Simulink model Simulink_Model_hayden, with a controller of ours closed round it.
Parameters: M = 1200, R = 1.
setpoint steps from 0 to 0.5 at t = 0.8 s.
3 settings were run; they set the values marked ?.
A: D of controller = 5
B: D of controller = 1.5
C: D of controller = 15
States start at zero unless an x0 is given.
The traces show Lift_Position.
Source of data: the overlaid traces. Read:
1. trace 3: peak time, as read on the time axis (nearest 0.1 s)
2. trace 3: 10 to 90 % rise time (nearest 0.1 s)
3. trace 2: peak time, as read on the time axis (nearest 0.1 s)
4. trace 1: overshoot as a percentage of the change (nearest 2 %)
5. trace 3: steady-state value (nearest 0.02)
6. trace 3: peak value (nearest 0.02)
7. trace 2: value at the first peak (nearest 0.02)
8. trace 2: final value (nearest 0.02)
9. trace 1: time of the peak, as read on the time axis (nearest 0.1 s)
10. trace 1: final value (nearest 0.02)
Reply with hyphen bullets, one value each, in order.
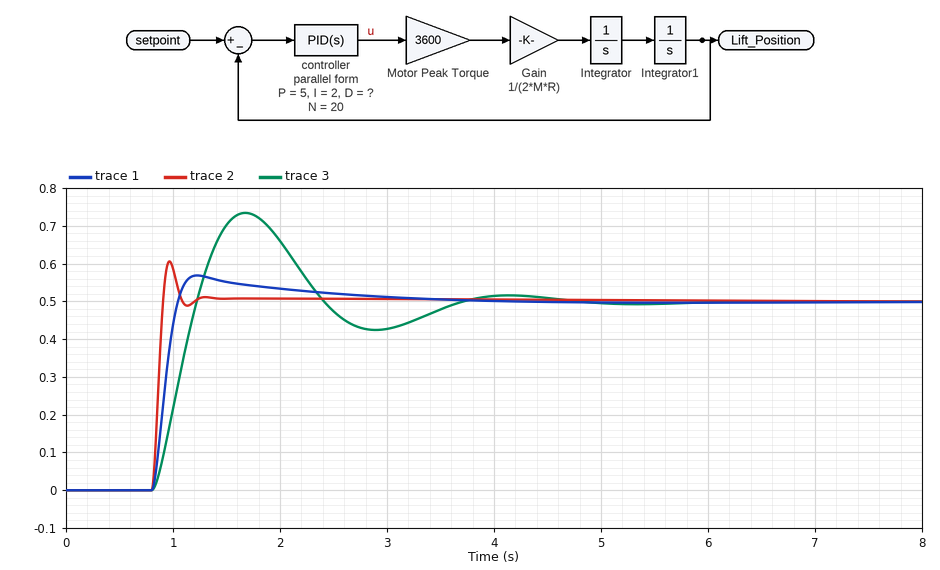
- 1.7 s
- 0.3 s
- 1.0 s
- 14 %
- 0.50
- 0.74
- 0.60
- 0.50
- 1.2 s
- 0.50
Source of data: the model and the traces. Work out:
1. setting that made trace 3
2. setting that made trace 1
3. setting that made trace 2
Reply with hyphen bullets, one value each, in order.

- B
- A
- C
